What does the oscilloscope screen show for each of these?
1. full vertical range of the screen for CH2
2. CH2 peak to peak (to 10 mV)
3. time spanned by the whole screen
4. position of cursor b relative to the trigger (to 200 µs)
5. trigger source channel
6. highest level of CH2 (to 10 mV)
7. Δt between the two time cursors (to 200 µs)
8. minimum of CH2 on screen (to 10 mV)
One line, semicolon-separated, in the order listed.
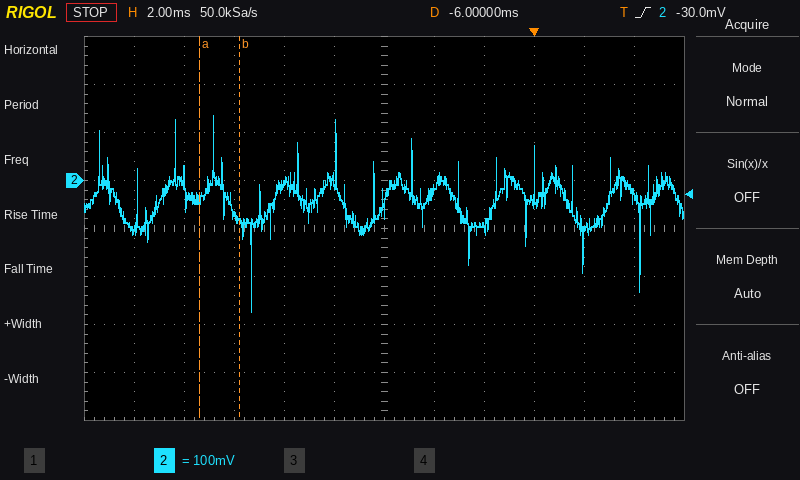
800 mV; 410 mV; 24 ms; -11.8 ms; CH2; 140 mV; 1.6 ms; -270 mV
